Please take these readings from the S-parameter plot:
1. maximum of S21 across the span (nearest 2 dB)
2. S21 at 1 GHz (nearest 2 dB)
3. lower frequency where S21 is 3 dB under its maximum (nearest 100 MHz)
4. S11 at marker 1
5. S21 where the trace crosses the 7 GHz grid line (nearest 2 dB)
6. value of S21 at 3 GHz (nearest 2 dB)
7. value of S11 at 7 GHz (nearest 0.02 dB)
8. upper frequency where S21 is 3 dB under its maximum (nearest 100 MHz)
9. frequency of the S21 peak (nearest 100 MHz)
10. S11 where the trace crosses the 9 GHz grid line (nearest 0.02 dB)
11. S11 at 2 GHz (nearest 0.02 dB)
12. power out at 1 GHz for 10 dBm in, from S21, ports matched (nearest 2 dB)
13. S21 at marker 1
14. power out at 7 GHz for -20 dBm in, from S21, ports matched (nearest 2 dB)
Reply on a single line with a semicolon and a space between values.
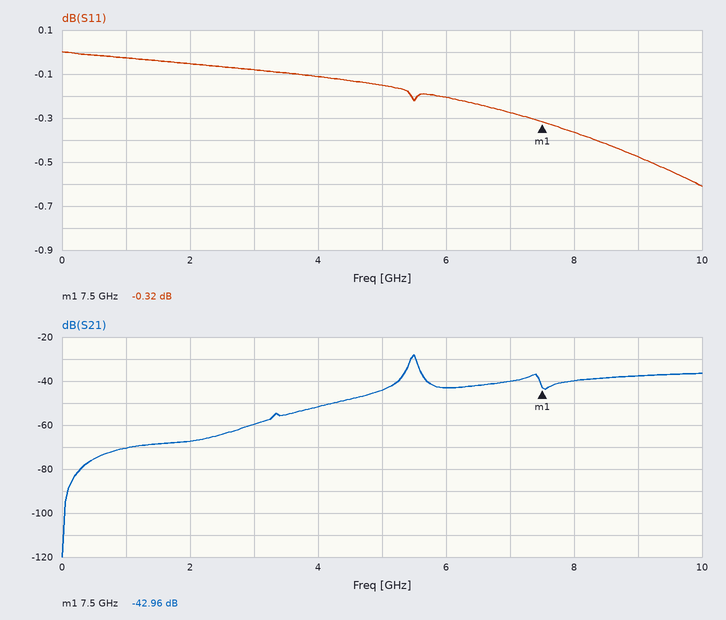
-28 dB; -70 dB; 5.4 GHz; -0.32 dB; -40 dB; -60 dB; -0.28 dB; 5.5 GHz; 5.5 GHz; -0.48 dB; -0.06 dB; -60 dBm; -42.96 dB; -60 dBm
